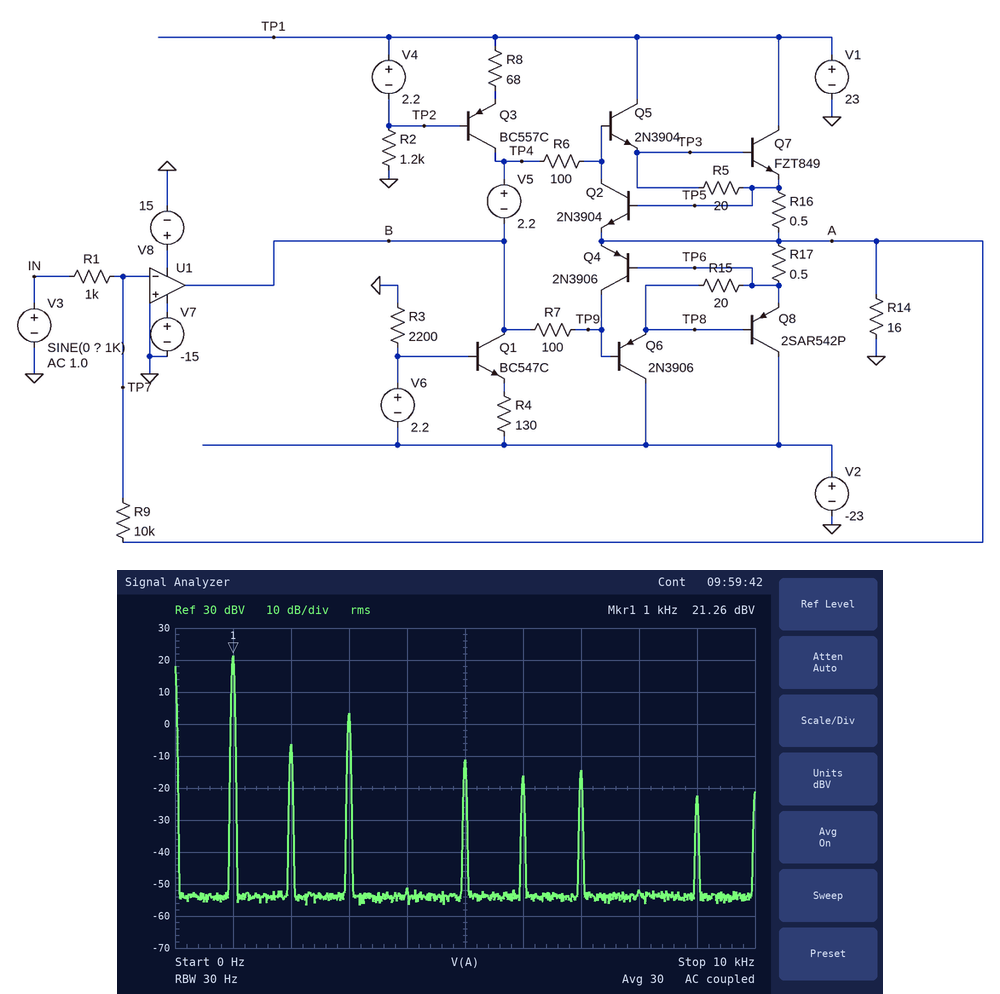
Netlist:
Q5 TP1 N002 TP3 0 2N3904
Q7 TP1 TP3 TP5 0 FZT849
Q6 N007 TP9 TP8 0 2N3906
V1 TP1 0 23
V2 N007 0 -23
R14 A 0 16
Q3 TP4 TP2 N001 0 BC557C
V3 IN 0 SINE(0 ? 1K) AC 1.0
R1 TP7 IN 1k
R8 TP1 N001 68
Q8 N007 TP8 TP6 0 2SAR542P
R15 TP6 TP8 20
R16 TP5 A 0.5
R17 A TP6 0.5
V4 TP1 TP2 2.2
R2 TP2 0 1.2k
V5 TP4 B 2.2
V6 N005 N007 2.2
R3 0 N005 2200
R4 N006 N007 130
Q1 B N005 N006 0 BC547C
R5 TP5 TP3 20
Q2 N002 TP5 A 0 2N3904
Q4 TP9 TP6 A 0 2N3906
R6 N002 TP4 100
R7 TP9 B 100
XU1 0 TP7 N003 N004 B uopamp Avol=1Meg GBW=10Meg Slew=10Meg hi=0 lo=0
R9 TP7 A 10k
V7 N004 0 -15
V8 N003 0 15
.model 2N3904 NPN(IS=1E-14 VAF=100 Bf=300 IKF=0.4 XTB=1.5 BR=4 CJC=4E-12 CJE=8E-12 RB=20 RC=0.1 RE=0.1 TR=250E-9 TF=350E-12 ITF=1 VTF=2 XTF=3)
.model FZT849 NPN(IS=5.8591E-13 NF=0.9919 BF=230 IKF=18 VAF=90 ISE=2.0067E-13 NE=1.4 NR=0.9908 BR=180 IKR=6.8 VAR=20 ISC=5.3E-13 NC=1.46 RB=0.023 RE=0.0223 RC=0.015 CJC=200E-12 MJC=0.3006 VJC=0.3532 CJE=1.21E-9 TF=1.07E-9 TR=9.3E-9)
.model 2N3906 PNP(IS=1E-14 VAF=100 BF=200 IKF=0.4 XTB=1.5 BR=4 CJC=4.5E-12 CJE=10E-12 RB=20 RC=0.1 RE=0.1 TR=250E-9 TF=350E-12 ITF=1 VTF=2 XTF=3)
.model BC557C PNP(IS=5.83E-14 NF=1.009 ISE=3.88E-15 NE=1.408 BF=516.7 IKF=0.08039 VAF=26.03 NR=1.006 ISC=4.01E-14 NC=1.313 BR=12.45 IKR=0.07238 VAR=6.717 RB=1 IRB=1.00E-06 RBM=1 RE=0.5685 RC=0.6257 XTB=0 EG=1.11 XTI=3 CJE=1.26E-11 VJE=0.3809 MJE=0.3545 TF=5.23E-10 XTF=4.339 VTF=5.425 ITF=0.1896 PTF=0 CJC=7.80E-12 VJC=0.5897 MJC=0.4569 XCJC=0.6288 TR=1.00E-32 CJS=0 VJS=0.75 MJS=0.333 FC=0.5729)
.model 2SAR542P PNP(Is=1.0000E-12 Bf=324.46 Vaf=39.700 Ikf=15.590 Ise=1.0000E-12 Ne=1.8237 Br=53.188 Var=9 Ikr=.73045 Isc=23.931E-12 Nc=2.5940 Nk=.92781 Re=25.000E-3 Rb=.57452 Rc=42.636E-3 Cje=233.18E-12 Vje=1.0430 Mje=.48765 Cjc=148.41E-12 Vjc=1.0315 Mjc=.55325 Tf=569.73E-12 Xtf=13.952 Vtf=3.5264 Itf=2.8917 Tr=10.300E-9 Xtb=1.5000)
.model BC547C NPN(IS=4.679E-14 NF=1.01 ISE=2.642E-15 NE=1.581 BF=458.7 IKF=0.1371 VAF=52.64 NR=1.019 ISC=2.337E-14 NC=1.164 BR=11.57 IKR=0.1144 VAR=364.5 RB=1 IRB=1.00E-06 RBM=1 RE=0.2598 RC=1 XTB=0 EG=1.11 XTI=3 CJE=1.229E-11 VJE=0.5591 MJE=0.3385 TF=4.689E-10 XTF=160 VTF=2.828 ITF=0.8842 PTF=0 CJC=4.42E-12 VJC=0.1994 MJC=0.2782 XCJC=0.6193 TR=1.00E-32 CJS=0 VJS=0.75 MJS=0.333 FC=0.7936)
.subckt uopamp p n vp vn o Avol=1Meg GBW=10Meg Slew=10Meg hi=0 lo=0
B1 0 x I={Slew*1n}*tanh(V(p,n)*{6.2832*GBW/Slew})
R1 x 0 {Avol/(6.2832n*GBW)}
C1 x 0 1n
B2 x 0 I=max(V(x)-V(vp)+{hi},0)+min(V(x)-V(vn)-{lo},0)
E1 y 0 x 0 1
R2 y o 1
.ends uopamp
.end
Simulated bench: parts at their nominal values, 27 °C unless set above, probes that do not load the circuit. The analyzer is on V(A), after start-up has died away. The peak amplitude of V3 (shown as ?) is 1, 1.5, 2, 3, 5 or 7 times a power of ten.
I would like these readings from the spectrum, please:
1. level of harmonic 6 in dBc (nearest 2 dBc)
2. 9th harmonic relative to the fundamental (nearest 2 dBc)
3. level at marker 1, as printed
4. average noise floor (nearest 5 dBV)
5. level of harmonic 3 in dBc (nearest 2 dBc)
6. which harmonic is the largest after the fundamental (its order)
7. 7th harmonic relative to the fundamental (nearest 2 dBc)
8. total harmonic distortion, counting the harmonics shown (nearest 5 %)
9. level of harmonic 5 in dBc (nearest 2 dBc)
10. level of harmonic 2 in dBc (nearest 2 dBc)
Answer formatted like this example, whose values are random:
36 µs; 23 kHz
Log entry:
-38 dBc; -44 dBc; 21.26 dBV; -55 dBV; -18 dBc; 3; -36 dBc; 15 %; -32 dBc; -28 dBc
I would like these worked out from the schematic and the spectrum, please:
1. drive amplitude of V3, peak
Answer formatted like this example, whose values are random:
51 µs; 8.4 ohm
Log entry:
2 V
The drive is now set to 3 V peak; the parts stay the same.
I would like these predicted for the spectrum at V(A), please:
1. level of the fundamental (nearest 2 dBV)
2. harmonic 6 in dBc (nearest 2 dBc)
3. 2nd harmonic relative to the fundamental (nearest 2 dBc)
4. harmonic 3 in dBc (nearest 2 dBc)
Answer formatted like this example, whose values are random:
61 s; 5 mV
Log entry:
22 dBV; -52 dBc; -30 dBc; -12 dBc
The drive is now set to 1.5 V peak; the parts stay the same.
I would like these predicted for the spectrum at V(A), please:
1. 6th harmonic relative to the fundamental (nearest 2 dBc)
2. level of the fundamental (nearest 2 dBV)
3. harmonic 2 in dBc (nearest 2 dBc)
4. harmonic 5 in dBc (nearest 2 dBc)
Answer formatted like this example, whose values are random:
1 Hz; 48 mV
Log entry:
-40 dBc; 20 dBV; -32 dBc; -38 dBc
